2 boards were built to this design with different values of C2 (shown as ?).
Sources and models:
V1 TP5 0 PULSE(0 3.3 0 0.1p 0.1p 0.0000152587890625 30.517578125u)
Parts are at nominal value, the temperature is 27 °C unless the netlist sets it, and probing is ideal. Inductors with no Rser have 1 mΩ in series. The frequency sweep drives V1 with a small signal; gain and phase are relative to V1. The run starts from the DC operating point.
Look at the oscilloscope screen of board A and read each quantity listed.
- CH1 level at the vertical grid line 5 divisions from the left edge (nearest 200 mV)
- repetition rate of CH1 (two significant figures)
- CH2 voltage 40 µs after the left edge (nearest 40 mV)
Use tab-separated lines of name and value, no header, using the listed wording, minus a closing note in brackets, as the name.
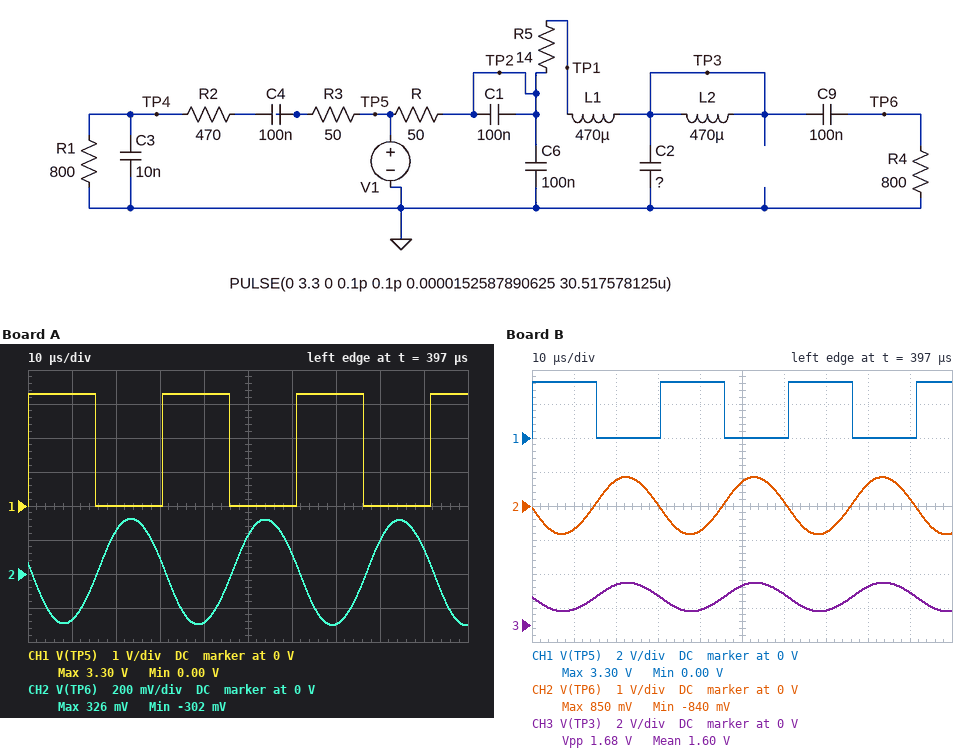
CH1 level at the vertical grid line 5 divisions from the left edge	0 V
repetition rate of CH1	33 kHz
CH2 voltage 40 µs after the left edge	-280 mV
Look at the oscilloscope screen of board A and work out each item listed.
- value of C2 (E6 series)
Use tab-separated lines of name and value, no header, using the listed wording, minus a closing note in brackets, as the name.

value of C2	330 nF
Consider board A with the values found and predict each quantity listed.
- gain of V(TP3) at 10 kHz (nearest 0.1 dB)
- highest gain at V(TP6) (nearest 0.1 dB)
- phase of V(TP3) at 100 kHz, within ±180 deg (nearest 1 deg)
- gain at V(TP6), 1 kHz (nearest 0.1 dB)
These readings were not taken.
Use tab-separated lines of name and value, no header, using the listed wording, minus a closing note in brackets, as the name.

gain of V(TP3) at 10 kHz	-3.8 dB
highest gain at V(TP6)	-2.3 dB
phase of V(TP3) at 100 kHz, within ±180 deg	112 deg
gain at V(TP6), 1 kHz	-7.2 dB
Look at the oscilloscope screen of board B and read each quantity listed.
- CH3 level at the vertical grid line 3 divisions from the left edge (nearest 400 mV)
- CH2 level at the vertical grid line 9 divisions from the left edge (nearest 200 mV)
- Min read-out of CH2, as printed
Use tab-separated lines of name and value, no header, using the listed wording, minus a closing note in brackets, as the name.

CH3 level at the vertical grid line 3 divisions from the left edge	1.6 V
CH2 level at the vertical grid line 9 divisions from the left edge	200 mV
Min read-out of CH2, as printed	-840 mV
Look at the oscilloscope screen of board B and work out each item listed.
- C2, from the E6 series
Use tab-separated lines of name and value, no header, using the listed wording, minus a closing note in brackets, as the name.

C2, from the E6 series	150 nF
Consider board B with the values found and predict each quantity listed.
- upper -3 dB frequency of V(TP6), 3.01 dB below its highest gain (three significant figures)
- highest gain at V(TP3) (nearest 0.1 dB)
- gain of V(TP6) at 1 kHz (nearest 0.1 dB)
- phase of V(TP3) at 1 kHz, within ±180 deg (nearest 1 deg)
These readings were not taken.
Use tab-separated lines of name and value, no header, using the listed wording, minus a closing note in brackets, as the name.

upper -3 dB frequency of V(TP6), 3.01 dB below its highest gain	27.4 kHz
highest gain at V(TP3)	0 dB
gain of V(TP6) at 1 kHz	-7.1 dB
phase of V(TP3) at 1 kHz, within ±180 deg	-7 deg
